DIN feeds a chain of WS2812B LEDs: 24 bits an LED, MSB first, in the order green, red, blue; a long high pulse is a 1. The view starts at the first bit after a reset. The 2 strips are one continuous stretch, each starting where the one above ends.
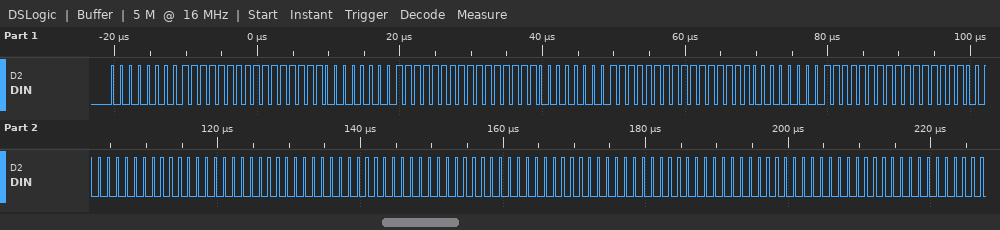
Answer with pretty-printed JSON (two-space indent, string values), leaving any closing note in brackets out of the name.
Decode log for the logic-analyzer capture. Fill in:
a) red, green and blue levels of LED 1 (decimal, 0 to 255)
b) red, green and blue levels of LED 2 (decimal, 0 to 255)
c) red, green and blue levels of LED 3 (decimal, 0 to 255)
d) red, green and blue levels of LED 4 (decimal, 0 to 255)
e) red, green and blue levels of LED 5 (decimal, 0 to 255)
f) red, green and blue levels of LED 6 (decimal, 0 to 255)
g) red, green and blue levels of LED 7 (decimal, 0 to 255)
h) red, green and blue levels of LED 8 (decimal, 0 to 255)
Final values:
{
  "red, green and blue levels of LED 1": "255, 0, 255",
  "red, green and blue levels of LED 2": "255, 0, 255",
  "red, green and blue levels of LED 3": "255, 0, 255",
  "red, green and blue levels of LED 4": "255, 0, 255",
  "red, green and blue levels of LED 5": "0, 0, 0",
  "red, green and blue levels of LED 6": "0, 0, 0",
  "red, green and blue levels of LED 7": "0, 0, 0",
  "red, green and blue levels of LED 8": "0, 0, 0"
}
